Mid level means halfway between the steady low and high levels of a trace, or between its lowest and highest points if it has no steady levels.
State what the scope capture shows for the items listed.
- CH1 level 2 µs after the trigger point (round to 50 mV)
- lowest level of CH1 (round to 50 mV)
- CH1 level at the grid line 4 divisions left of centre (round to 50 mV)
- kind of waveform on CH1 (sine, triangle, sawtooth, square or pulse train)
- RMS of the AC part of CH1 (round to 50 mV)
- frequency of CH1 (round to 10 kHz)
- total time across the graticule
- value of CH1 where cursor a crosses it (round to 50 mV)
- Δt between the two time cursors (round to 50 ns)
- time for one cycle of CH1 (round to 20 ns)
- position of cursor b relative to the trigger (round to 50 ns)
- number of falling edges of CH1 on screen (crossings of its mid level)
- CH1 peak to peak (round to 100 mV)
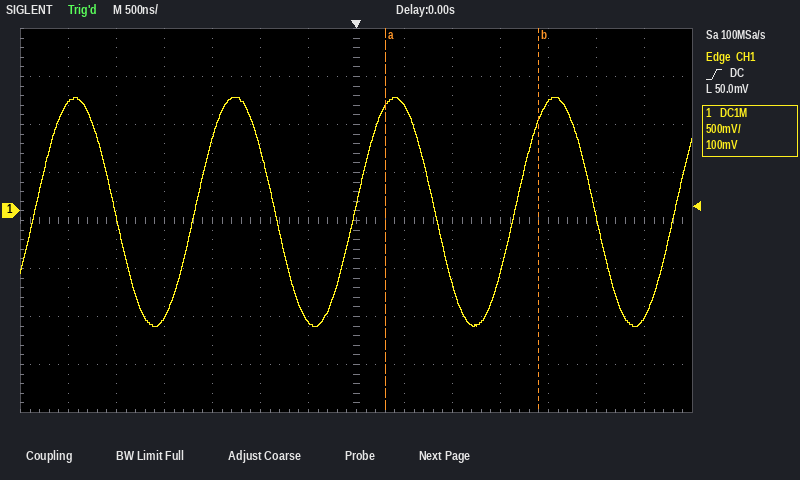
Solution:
1.15 V
-1.20 V
-1.10 V
sine
850 mV
600 kHz
7 µs
1.10 V
1.60 µs
1.66 µs
+1.90 µs
4
2.40 V
